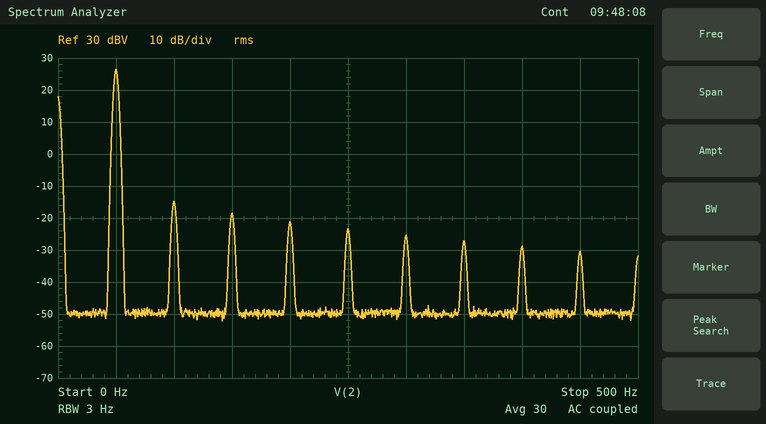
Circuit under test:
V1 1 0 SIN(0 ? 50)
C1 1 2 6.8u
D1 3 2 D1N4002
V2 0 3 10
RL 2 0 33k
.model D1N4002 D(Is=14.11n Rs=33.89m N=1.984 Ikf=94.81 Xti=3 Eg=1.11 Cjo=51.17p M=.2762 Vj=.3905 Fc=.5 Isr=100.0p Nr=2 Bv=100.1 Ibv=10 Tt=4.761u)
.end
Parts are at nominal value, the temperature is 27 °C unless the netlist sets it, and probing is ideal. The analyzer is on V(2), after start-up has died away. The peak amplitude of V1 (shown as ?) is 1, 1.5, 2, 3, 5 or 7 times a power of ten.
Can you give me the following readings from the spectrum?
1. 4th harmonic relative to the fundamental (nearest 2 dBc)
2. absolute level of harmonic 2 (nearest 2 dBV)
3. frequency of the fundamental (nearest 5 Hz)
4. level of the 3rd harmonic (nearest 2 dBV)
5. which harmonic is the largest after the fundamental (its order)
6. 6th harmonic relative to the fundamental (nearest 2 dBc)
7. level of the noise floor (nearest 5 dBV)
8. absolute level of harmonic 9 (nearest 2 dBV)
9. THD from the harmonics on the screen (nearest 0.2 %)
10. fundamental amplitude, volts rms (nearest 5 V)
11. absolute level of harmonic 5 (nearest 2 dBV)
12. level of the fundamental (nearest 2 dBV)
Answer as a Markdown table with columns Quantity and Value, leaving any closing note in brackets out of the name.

| Quantity | Value |
|---|---|
| 4th harmonic relative to the fundamental | -48 dBc |
| absolute level of harmonic 2 | -14 dBV |
| frequency of the fundamental | 50 Hz |
| level of the 3rd harmonic | -18 dBV |
| which harmonic is the largest after the fundamental | 2 |
| 6th harmonic relative to the fundamental | -52 dBc |
| level of the noise floor | -50 dBV |
| absolute level of harmonic 9 | -30 dBV |
| THD from the harmonics on the screen | 1.2 % |
| fundamental amplitude, volts rms | 20 V |
| absolute level of harmonic 5 | -24 dBV |
| level of the fundamental | 26 dBV |
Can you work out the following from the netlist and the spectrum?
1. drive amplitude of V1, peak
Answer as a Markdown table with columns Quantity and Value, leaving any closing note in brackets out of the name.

| Quantity | Value |
|---|---|
| drive amplitude of V1, peak | 30 V |
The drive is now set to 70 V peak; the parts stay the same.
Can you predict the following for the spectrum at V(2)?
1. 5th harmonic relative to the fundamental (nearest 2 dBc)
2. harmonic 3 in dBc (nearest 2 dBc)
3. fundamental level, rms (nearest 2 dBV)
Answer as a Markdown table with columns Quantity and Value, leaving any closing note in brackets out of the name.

| Quantity | Value |
|---|---|
| 5th harmonic relative to the fundamental | -30 dBc |
| harmonic 3 in dBc | -20 dBc |
| fundamental level, rms | 32 dBV |
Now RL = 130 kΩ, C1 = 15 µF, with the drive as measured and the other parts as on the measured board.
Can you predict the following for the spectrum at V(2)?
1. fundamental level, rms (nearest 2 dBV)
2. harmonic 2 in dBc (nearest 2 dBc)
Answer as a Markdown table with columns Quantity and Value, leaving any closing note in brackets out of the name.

| Quantity | Value |
|---|---|
| fundamental level, rms | 26 dBV |
| harmonic 2 in dBc | -60 dBc |
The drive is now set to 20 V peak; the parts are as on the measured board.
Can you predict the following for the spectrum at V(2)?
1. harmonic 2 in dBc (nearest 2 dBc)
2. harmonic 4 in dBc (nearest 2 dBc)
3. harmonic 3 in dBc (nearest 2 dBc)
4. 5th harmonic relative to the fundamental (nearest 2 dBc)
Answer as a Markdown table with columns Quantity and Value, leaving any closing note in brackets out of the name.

| Quantity | Value |
|---|---|
| harmonic 2 in dBc | -44 dBc |
| harmonic 4 in dBc | -50 dBc |
| harmonic 3 in dBc | -48 dBc |
| 5th harmonic relative to the fundamental | -52 dBc |
